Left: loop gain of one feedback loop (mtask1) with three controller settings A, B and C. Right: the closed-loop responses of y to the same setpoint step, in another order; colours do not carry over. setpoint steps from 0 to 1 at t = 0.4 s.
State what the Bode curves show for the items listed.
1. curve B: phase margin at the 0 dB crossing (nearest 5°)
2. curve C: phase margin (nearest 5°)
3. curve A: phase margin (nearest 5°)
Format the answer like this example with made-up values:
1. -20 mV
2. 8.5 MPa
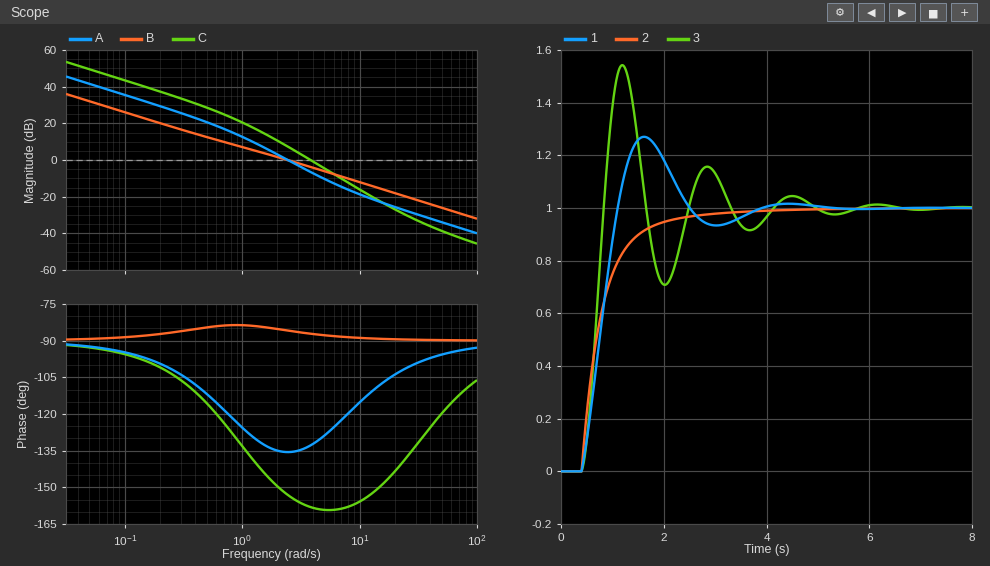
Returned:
1. 95°
2. 20°
3. 45°
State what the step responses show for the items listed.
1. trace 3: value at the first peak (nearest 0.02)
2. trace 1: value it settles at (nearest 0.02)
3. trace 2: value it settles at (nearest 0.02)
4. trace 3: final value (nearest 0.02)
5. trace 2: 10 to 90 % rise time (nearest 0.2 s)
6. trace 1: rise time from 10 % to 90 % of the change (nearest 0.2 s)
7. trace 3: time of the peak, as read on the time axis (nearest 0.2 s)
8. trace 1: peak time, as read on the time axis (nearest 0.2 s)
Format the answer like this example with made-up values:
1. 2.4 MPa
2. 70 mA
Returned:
1. 1.54
2. 1.00
3. 1.00
4. 1.00
5. 1.0 s
6. 0.6 s
7. 1.2 s
8. 1.6 s
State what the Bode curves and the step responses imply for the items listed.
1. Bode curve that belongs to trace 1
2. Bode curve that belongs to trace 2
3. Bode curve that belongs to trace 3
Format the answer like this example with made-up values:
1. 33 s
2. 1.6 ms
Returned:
1. A
2. B
3. C
